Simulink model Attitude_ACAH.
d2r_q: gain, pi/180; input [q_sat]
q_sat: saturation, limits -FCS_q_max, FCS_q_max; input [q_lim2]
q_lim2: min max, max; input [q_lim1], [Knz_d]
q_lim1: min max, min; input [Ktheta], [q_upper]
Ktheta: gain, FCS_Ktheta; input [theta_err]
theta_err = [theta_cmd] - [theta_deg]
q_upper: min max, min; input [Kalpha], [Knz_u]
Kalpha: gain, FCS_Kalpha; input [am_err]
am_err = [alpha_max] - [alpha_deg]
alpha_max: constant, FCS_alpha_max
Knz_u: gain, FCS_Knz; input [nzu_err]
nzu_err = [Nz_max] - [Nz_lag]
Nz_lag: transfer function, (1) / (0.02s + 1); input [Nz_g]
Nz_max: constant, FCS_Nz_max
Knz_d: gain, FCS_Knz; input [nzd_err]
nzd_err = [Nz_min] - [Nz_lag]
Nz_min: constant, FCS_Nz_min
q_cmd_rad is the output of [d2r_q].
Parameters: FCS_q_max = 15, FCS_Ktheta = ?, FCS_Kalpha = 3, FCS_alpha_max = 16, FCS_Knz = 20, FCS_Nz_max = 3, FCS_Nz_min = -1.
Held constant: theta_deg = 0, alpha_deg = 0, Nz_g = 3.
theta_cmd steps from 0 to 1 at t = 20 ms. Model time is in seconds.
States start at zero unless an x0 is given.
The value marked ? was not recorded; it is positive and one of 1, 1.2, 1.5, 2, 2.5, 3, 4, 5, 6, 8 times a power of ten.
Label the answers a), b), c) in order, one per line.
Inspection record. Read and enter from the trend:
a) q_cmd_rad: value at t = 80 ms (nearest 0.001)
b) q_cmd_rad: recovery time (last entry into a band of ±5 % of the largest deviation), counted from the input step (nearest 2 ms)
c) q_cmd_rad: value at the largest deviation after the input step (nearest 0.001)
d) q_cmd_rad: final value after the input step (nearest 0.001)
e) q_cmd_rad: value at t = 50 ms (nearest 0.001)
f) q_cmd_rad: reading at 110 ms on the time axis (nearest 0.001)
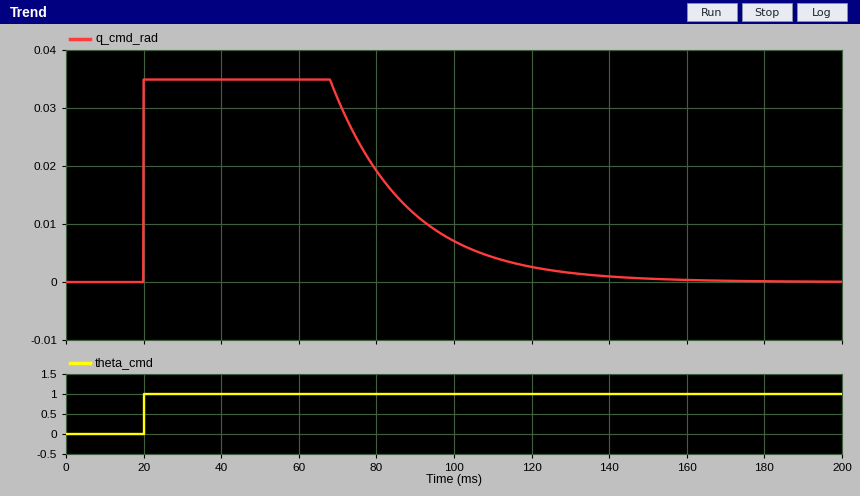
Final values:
a) 0.019
b) 108 ms
c) 0.035
d) 0.000
e) 0.035
f) 0.004
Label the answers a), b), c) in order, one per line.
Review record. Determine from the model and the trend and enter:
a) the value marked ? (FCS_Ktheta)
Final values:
a) 2
